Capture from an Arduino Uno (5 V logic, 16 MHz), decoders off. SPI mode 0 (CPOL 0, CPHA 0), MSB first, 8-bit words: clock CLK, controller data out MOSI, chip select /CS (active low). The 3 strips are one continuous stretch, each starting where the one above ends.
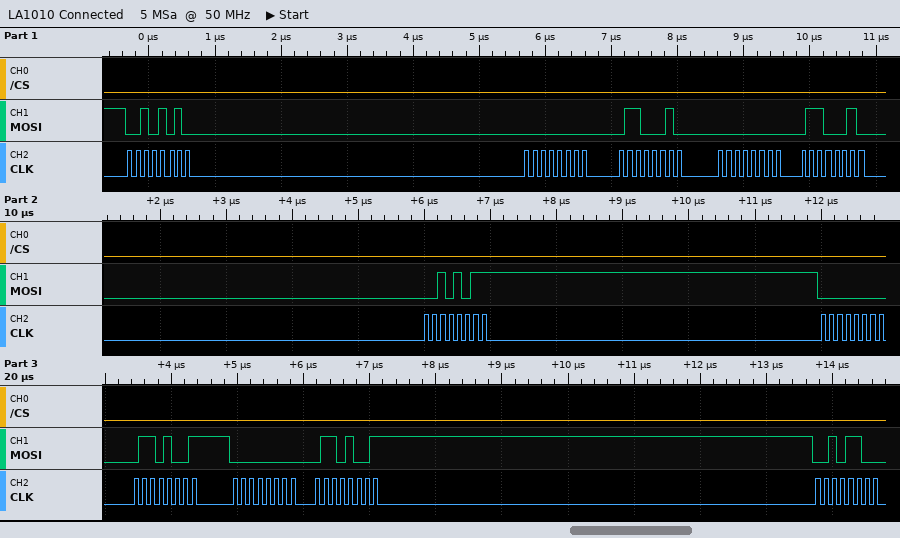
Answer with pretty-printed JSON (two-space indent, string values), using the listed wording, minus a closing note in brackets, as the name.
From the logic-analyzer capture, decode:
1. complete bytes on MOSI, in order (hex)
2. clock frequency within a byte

{
  "complete bytes on MOSI, in order": "2A 00 62 00 62 2B 00 69 00 69 2C",
  "clock frequency within a byte": "8 MHz"
}
